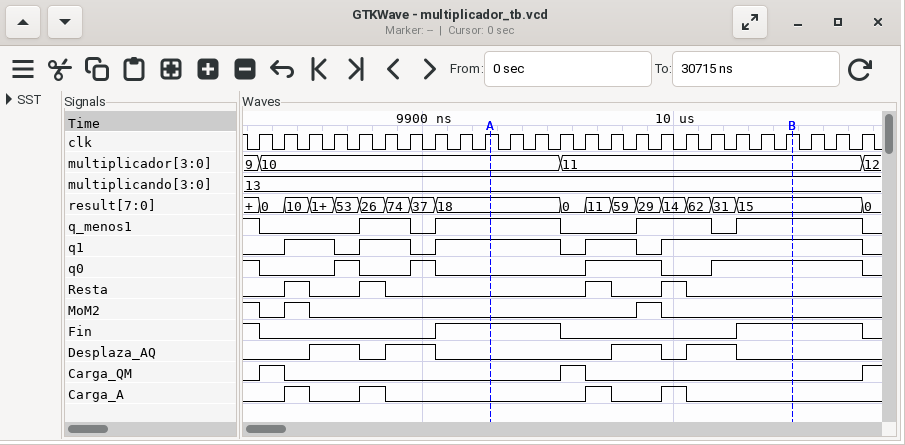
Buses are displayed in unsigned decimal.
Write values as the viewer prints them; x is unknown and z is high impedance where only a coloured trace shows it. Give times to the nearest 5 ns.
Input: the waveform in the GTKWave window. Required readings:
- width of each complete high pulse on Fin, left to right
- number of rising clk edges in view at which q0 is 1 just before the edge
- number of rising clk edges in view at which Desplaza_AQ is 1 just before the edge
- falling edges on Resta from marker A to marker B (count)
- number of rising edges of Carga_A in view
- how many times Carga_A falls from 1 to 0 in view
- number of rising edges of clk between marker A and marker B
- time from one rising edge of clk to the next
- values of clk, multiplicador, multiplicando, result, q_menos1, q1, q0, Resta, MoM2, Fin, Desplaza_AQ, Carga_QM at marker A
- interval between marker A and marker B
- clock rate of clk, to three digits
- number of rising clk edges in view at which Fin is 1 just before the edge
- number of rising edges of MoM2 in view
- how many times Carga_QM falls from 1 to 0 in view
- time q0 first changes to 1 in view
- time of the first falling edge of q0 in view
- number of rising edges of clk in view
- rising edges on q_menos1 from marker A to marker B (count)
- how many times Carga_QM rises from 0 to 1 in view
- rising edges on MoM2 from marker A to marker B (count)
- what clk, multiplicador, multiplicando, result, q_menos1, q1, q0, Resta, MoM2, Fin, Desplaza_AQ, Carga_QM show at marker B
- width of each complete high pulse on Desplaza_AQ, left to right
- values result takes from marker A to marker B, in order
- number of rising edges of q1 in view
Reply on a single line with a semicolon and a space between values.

50 ns, 50 ns; 12; 8; 2; 4; 4; 12; 10 ns; clk=1, multiplicador=10, multiplicando=13, result=18, q_menos1=1, q1=1, q0=0, Resta=0, MoM2=0, Fin=1, Desplaza_AQ=0, Carga_QM=0; 120 ns; 100 MHz; 11; 2; 2; 9865 ns; 9835 ns; 25; 2; 3; 1; clk=1, multiplicador=11, multiplicando=13, result=15, q_menos1=1, q1=1, q0=1, Resta=0, MoM2=0, Fin=1, Desplaza_AQ=0, Carga_QM=0; 20 ns, 20 ns, 20 ns, 20 ns; 18, 0, 11, 59, 29, 14, 62, 31, 15; 5
